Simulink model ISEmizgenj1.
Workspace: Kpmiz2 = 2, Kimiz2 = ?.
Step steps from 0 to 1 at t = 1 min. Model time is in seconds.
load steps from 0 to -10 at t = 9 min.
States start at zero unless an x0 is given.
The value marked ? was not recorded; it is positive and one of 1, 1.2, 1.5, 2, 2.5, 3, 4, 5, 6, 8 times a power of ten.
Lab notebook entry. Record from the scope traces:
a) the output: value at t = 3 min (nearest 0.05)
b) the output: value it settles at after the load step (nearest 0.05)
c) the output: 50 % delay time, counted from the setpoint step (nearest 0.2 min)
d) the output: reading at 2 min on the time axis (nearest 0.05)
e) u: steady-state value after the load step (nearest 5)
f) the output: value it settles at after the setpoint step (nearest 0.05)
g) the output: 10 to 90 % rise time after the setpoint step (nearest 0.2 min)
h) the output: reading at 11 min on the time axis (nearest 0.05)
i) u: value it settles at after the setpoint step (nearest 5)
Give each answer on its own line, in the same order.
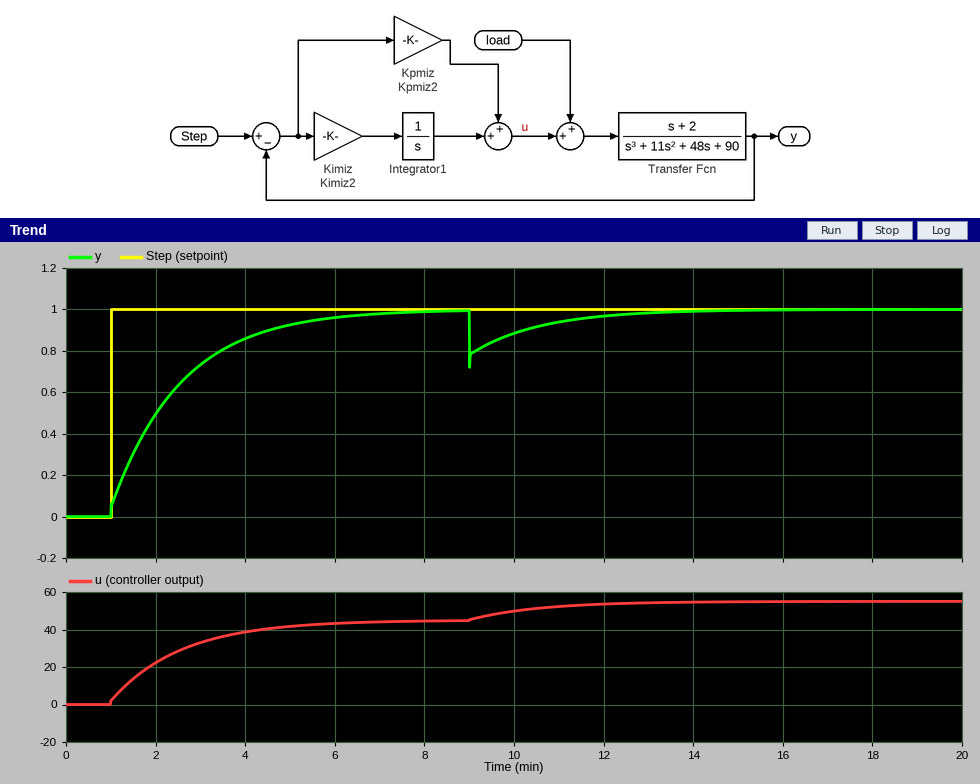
0.75
1.00
1.0 min
0.50
55
1.00
3.4 min
0.95
45
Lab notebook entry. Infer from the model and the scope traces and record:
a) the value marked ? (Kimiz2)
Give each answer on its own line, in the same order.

0.5
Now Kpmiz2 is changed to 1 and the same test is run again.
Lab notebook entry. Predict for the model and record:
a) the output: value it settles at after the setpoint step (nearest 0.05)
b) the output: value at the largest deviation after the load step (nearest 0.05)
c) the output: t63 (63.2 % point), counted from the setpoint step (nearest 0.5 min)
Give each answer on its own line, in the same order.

1.00
0.70
1.5 min
